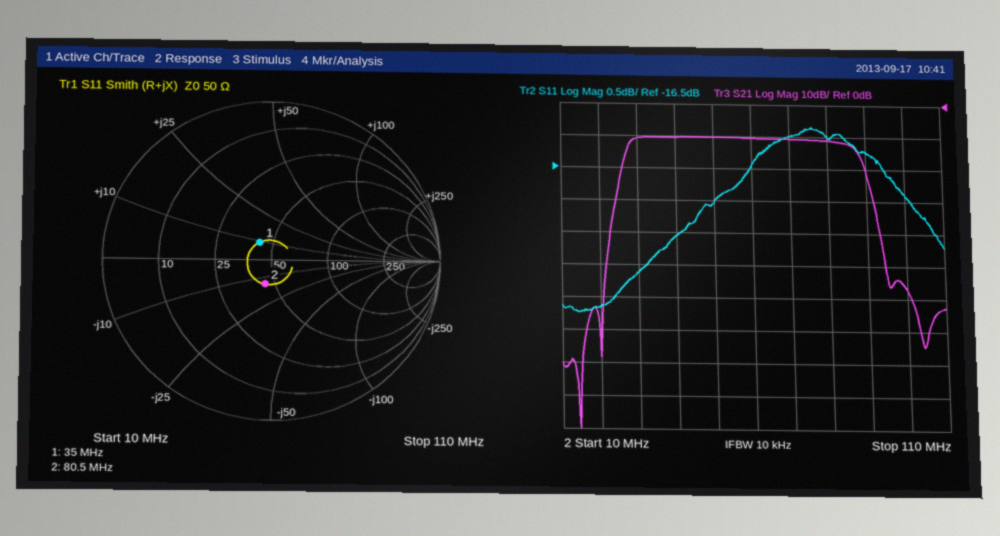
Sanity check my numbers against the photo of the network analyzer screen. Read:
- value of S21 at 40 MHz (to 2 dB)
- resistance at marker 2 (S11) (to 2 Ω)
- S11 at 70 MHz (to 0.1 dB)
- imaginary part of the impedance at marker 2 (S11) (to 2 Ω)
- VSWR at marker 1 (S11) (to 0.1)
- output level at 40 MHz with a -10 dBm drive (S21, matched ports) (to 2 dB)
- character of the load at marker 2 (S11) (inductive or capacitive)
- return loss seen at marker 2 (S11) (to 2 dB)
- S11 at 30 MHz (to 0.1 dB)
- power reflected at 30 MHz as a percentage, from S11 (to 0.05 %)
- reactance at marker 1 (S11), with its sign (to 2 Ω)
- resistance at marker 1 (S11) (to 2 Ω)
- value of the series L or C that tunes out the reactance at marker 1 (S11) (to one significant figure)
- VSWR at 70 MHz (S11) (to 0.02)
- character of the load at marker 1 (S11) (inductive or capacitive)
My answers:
-10 dB
44 Ω
-16.0 dB
-14 Ω
1.3
-20 dBm
capacitive
16 dB
-18.1 dB
1.55 %
+10 Ω
42 Ω
500 pF
1.38
inductive
